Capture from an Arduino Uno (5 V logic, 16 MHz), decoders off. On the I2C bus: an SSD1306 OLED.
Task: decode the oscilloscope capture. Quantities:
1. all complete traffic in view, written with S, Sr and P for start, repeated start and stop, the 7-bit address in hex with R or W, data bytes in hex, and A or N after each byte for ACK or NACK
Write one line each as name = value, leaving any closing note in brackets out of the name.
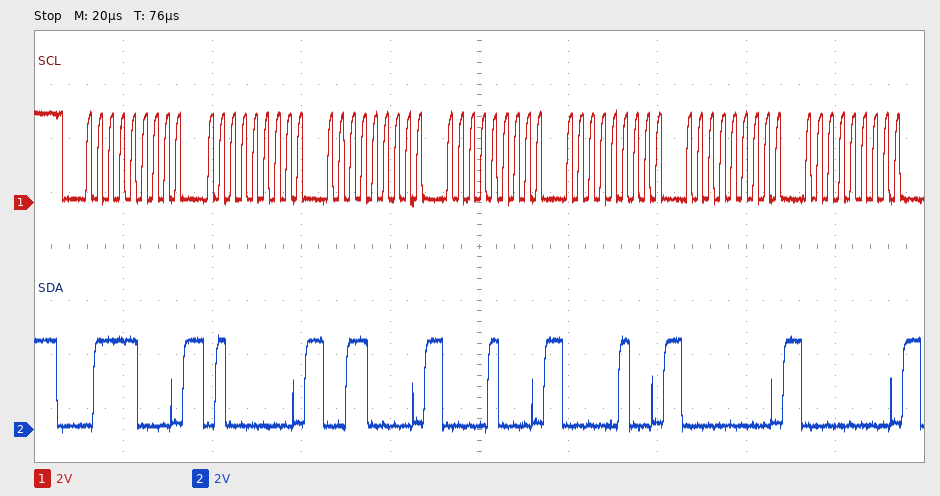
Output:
all complete traffic in view, written with S, Sr and P for start, repeated start and stop, the 7-bit address in hex with R or W, data bytes in hex, and A or N after each byte for ACK or NACK = S 3CW A 40 A 30 A 08 A 04 A 00 A 00 A
